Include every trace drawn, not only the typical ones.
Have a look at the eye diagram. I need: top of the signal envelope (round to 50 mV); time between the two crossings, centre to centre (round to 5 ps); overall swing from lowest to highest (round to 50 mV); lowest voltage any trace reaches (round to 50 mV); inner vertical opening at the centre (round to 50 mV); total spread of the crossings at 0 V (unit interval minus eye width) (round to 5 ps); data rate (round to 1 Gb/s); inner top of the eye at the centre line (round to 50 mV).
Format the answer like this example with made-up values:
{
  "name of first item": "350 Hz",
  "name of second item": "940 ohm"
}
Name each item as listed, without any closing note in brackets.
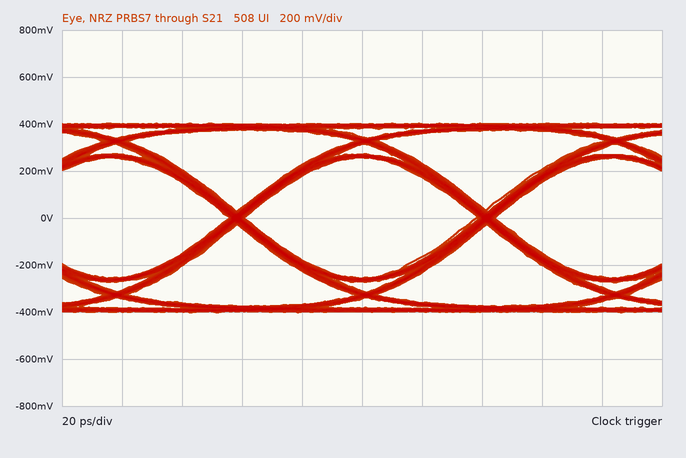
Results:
{
  "top of the signal envelope": "400 mV",
  "time between the two crossings, centre to centre": "85 ps",
  "overall swing from lowest to highest": "800 mV",
  "lowest voltage any trace reaches": "-400 mV",
  "inner vertical opening at the centre": "500 mV",
  "total spread of the crossings at 0 V (unit interval minus eye width)": "5 ps",
  "data rate": "12 Gb/s",
  "inner top of the eye at the centre line": "250 mV"
}
